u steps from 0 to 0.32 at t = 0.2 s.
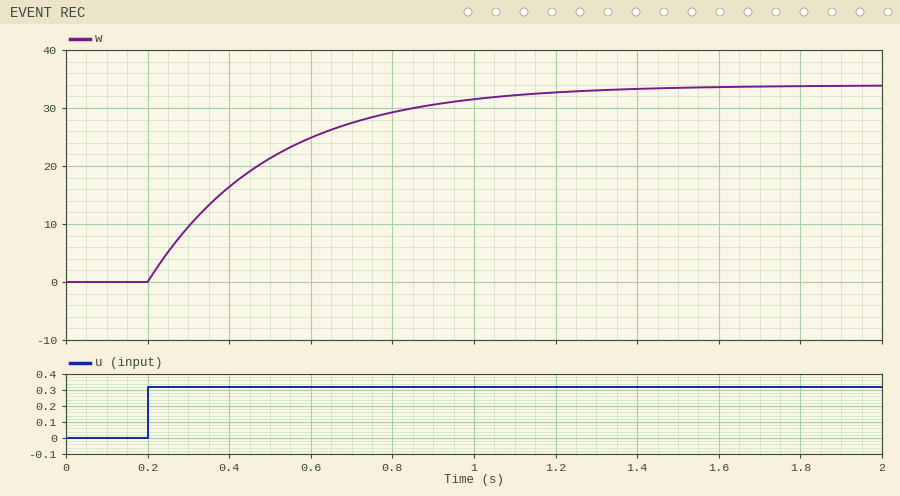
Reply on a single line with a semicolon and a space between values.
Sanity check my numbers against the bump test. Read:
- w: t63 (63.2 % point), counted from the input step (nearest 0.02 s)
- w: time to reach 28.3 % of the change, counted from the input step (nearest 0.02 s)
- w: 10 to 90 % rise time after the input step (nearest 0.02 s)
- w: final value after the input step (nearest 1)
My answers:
0.30 s; 0.10 s; 0.66 s; 34
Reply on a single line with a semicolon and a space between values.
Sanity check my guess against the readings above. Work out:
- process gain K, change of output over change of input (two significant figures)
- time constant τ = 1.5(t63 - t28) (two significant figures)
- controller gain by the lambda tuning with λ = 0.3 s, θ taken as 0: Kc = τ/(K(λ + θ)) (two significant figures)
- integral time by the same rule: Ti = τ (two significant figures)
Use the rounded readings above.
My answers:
110; 0.30 s; 0.0091; 0.30 s
